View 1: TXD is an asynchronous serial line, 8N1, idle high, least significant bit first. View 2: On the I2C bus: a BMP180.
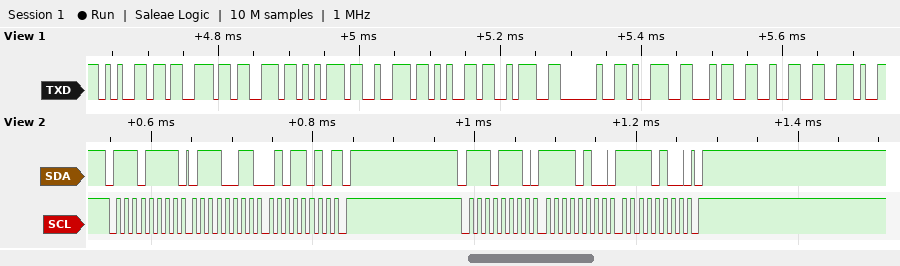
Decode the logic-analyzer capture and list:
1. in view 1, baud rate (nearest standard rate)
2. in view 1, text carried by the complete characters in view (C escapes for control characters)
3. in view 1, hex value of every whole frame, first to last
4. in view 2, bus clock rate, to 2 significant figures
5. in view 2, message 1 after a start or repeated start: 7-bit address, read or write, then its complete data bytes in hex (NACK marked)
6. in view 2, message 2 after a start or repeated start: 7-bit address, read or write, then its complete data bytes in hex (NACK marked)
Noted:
115200 baud
"essure: 942."
65 73 73 75 72 65 3A 20 39 34 32 2E
100 kHz
0x77 read: 73 5A NACK
0x77 write: F4 F4
